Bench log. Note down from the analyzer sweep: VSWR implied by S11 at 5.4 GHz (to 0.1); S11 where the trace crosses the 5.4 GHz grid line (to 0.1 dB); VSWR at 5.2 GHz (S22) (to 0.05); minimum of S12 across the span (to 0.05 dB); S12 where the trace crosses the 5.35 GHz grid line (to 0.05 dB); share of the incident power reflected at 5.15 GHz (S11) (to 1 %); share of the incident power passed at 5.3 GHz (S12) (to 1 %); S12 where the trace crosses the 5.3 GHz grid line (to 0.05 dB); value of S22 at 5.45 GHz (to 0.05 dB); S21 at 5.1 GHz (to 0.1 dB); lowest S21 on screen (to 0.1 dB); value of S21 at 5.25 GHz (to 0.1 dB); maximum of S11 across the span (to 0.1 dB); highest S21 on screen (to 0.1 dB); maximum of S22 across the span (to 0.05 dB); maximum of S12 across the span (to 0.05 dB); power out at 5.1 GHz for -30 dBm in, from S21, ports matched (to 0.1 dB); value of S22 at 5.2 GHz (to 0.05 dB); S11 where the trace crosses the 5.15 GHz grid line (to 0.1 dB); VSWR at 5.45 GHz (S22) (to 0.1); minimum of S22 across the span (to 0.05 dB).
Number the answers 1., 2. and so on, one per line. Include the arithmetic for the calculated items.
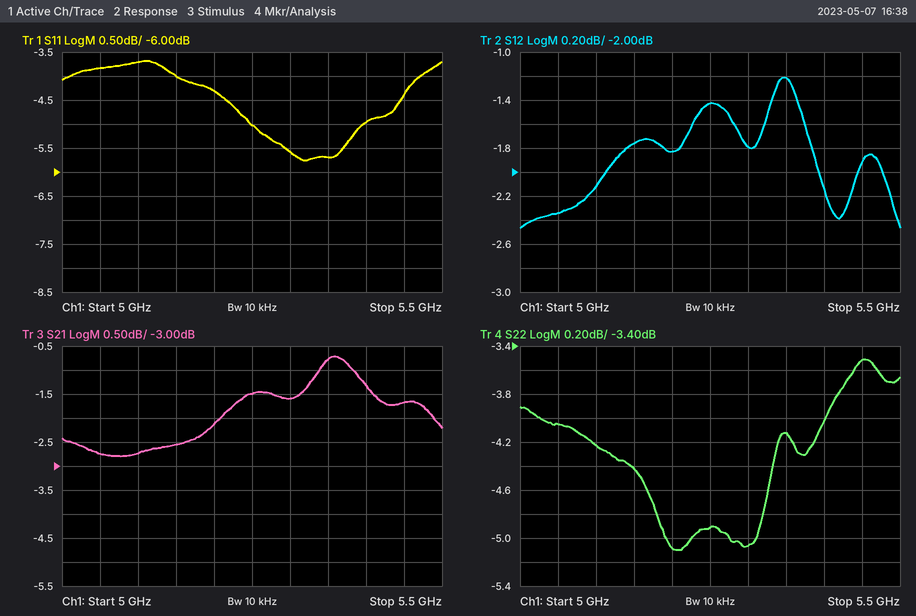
1. |Γ| = 10^(-5/20) = 0.5623; VSWR = (1 + 0.5623)/(1 − 0.5623) ≈ 3.6
2. -5.0 dB
3. |Γ| = 10^(-5.1/20) = 0.5559; VSWR = (1 + 0.5559)/(1 − 0.5559) ≈ 3.50
4. -2.45 dB
5. -1.20 dB
6. 10^(-4/10) ≈ 40 %
7. 10^(-1.8/10) ≈ 66 %
8. -1.80 dB
9. -3.50 dB
10. -2.7 dB
11. -2.8 dB
12. -1.5 dB
13. -3.7 dB
14. -0.7 dB
15. -3.50 dB
16. -1.20 dB
17. -30 dBm + (-2.7 dB) = -32.7 dBm
18. -5.10 dB
19. -4.0 dB
20. |Γ| = 10^(-3.5/20) = 0.6683; VSWR = (1 + 0.6683)/(1 − 0.6683) ≈ 5.0
21. -5.10 dB
